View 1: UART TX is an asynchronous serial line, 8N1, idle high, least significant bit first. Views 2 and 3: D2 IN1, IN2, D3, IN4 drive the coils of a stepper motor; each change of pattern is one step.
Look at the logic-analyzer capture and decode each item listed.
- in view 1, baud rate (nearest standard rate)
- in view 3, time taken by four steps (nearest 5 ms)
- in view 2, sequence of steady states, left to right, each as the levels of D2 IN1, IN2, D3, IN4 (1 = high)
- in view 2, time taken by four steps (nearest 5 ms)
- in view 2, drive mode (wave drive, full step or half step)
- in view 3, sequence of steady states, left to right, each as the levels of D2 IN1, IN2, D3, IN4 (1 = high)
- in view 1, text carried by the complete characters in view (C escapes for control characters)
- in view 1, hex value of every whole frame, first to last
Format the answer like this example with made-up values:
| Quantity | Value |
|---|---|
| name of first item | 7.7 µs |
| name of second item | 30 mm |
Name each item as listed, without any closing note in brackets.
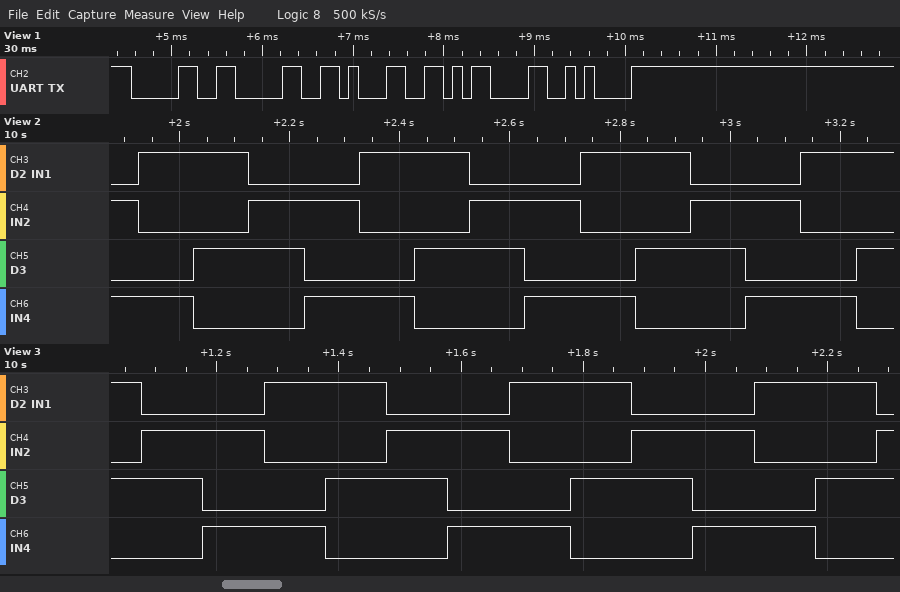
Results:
| Quantity | Value |
|---|---|
| in view 1, baud rate | 9600 baud |
| in view 3, time taken by four steps | 400 ms |
| in view 2, sequence of steady states, left to right, each as the levels of D2 IN1, IN2, D3, IN4 | 0101 1001 1010 0110 0101 1001 1010 0110 0101 1001 1010 0110 0101 1001 1010 |
| in view 2, time taken by four steps | 400 ms |
| in view 2, drive mode | full step |
| in view 3, sequence of steady states, left to right, each as the levels of D2 IN1, IN2, D3, IN4 | 1010 0110 0101 1001 1010 0110 0101 1001 1010 0110 0101 1001 1010 0110 |
| in view 1, text carried by the complete characters in view | "001\r\n" |
| in view 1, hex value of every whole frame, first to last | 30 30 31 0D 0A |
